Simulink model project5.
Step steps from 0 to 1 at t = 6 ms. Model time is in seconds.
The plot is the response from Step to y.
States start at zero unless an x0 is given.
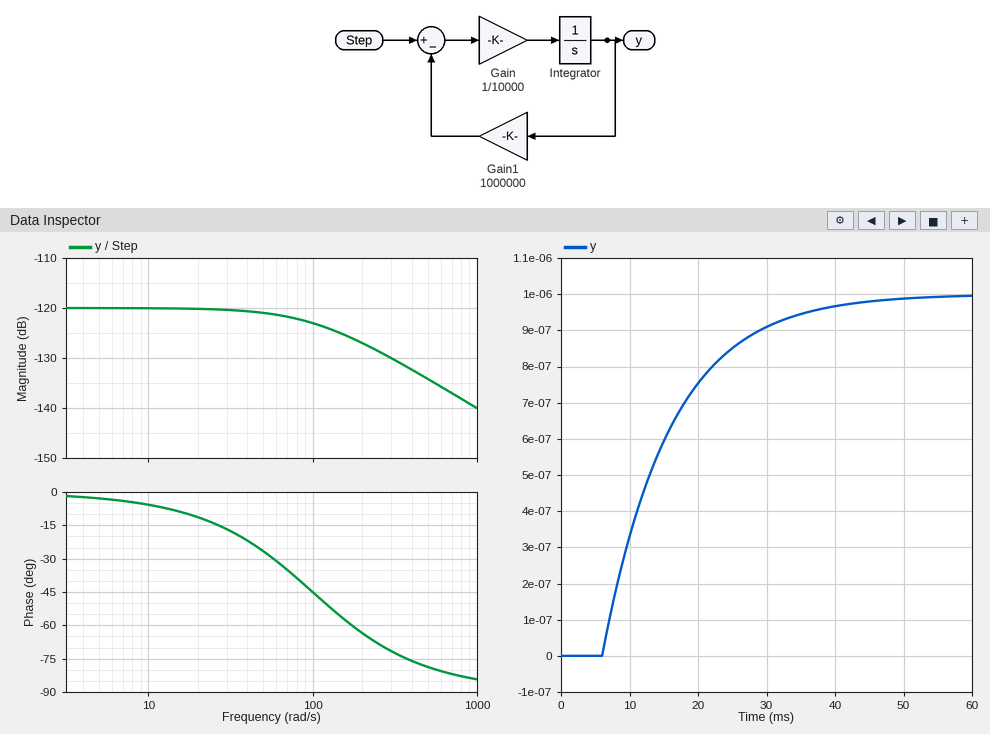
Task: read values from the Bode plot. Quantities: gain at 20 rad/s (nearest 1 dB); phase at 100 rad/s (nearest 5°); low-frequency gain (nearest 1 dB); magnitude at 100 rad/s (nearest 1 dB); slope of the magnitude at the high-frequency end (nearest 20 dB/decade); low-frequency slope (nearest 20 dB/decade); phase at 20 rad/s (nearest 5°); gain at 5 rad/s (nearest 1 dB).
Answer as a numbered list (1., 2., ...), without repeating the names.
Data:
1. -120 dB
2. -45°
3. -120 dB
4. -123 dB
5. -20 dB/decade
6. 0 dB/decade
7. -10°
8. -120 dB
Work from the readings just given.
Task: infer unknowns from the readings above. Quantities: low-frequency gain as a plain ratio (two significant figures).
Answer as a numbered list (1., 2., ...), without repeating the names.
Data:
1. 0.0000010
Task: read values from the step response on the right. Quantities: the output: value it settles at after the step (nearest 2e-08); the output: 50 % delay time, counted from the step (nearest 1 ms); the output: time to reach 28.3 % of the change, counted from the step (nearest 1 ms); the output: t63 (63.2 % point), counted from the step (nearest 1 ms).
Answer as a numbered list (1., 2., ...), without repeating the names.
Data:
1. 0.00000100
2. 7 ms
3. 3 ms
4. 10 ms
